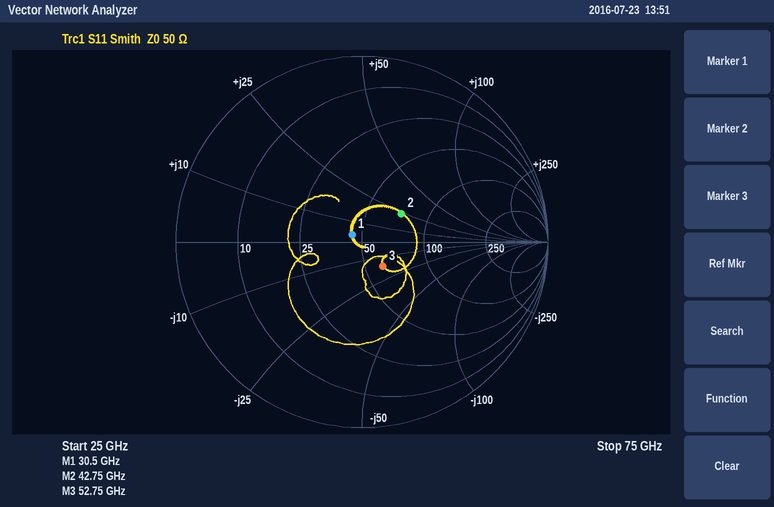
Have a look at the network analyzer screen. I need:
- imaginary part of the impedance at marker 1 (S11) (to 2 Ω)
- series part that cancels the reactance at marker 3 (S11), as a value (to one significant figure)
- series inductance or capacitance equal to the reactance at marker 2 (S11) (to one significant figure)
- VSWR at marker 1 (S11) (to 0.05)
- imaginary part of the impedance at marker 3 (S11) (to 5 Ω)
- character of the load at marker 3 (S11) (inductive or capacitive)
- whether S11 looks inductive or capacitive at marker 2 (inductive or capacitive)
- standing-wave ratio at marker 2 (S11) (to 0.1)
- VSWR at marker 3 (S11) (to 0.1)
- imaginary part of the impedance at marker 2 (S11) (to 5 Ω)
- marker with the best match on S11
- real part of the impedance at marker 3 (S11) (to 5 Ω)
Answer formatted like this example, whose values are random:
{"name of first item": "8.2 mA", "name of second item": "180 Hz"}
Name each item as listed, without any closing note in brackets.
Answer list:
{"imaginary part of the impedance at marker 1 (S11)": "+4 Ω", "series part that cancels the reactance at marker 3 (S11), as a value": "50 pH", "series inductance or capacitance equal to the reactance at marker 2 (S11)": "90 pH", "VSWR at marker 1 (S11)": "1.15", "imaginary part of the impedance at marker 3 (S11)": "-15 Ω", "character of the load at marker 3 (S11)": "capacitive", "whether S11 looks inductive or capacitive at marker 2": "inductive", "standing-wave ratio at marker 2 (S11)": "1.7", "VSWR at marker 3 (S11)": "1.4", "imaginary part of the impedance at marker 2 (S11)": "+25 Ω", "marker with the best match on S11": "marker 1", "real part of the impedance at marker 3 (S11)": "60 Ω"}
